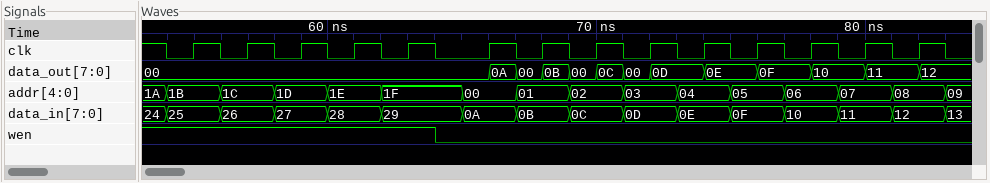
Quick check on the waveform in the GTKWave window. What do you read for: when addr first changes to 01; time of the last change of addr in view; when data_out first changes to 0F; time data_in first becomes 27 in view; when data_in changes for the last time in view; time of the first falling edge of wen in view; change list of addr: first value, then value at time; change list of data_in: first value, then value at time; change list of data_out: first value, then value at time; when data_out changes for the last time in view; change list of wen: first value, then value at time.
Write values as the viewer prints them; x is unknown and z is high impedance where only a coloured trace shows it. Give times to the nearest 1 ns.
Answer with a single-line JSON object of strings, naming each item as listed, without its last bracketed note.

{"when addr first changes to 01": "67 ns", "time of the last change of addr in view": "83 ns", "when data_out first changes to 0F": "76 ns", "time data_in first becomes 27 in view": "58 ns", "when data_in changes for the last time in view": "83 ns", "time of the first falling edge of wen in view": "64 ns", "change list of addr: first value, then value at time": "1A, 1B at 54 ns, 1C at 56 ns, 1D at 58 ns, 1E at 60 ns, 1F at 62 ns, 00 at 65 ns, 01 at 67 ns, 02 at 69 ns, 03 at 71 ns, 04 at 73 ns, 05 at 75 ns, 06 at 77 ns, 07 at 79 ns, 08 at 81 ns, 09 at 83 ns", "change list of data_in: first value, then value at time": "24, 25 at 54 ns, 26 at 56 ns, 27 at 58 ns, 28 at 60 ns, 29 at 62 ns, 0A at 65 ns, 0B at 67 ns, 0C at 69 ns, 0D at 71 ns, 0E at 73 ns, 0F at 75 ns, 10 at 77 ns, 11 at 79 ns, 12 at 81 ns, 13 at 83 ns", "change list of data_out: first value, then value at time": "00, 0A at 66 ns, 00 at 67 ns, 0B at 68 ns, 00 at 69 ns, 0C at 70 ns, 00 at 71 ns, 0D at 72 ns, 0E at 74 ns, 0F at 76 ns, 10 at 78 ns, 11 at 80 ns, 12 at 82 ns", "when data_out changes for the last time in view": "82 ns", "change list of wen: first value, then value at time": "1, 0 at 64 ns"}
